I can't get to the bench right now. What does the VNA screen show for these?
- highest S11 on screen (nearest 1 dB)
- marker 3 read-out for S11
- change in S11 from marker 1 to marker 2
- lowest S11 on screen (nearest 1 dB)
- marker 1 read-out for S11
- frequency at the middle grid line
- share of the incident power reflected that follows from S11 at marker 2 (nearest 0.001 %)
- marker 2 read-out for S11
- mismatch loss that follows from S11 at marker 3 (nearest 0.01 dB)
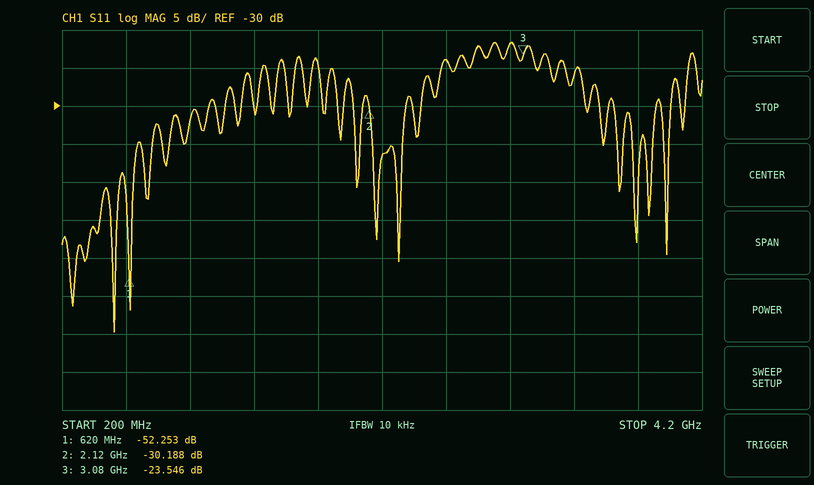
-22 dB
-23.546 dB
22.065 dB
-60 dB
-52.253 dB
2.2 GHz
0.096 %
-30.188 dB
0.02 dB
